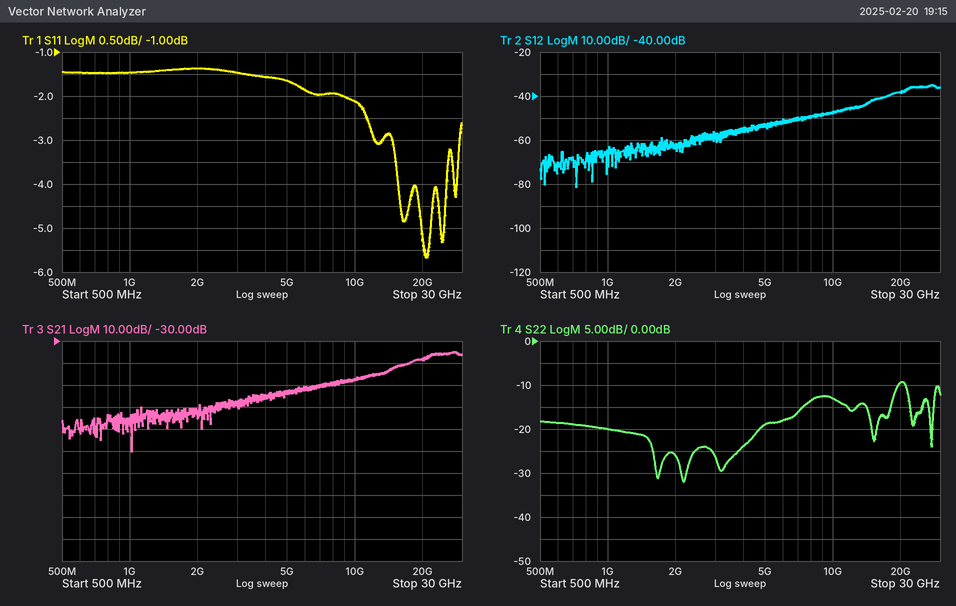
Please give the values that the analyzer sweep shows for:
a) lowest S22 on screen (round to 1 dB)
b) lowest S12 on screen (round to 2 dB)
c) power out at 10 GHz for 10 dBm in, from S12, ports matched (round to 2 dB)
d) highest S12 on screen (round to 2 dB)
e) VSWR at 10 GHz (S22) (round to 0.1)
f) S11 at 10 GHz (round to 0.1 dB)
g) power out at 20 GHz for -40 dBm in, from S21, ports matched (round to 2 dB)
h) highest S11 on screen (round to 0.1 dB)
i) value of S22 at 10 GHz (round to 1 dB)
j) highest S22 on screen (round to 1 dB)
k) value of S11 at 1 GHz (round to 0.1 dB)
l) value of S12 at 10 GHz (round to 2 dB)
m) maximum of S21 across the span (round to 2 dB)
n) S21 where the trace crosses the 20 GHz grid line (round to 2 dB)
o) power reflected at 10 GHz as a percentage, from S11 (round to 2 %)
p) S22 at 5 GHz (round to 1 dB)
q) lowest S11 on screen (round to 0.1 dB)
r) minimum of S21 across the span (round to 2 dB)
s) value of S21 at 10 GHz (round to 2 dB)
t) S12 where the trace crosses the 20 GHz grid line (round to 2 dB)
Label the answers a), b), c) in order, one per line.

a) -32 dB
b) -82 dB
c) -38 dBm
d) -34 dB
e) 1.6
f) -2.1 dB
g) -78 dBm
h) -1.4 dB
i) -13 dB
j) -9 dB
k) -1.5 dB
l) -48 dB
m) -34 dB
n) -38 dB
o) 62 %
p) -19 dB
q) -5.7 dB
r) -80 dB
s) -48 dB
t) -38 dB
